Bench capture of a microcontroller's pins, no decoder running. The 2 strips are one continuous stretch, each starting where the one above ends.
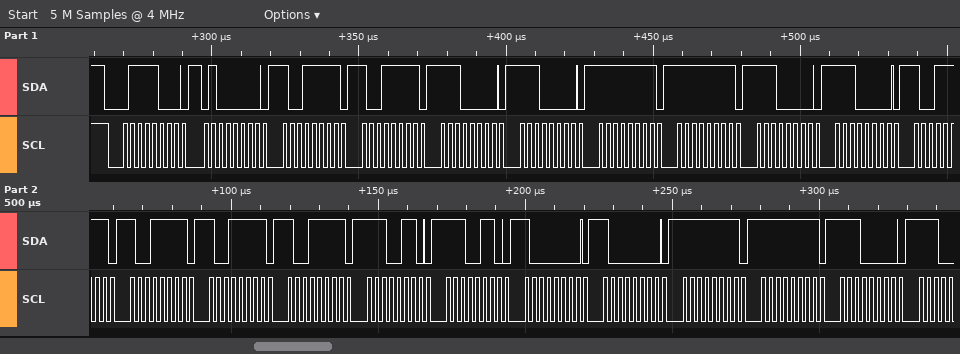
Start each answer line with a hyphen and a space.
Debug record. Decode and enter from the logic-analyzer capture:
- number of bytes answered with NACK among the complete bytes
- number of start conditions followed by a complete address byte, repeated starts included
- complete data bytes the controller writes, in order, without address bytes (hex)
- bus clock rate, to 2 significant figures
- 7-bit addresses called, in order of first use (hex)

- 0
- 1
- 40 9F 9F E0 E0 FF FF E0 E0 9F 9F 9F 9F E6 E6 80 80 FF FF E0
- 400 kHz
- 0x3C
